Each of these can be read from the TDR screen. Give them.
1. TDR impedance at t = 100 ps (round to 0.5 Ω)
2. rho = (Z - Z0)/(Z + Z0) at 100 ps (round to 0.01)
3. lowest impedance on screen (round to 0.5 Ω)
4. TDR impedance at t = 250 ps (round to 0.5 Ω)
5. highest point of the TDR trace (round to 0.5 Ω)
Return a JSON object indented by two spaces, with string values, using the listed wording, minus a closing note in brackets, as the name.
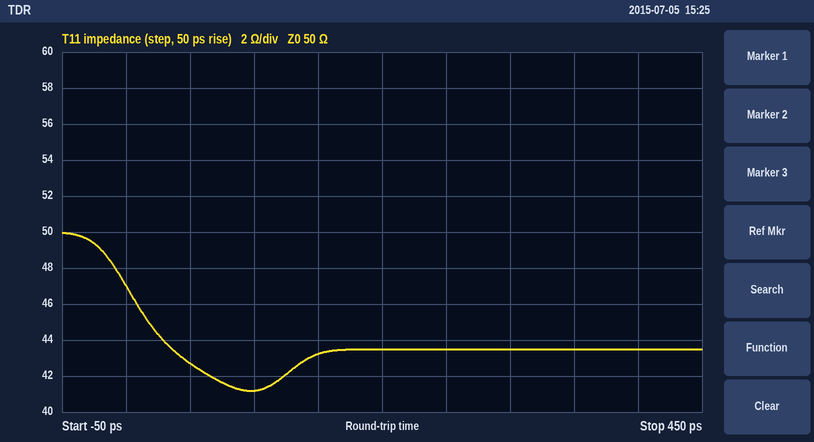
{
  "TDR impedance at t = 100 ps": "41.0 Ω",
  "rho = (Z - Z0)/(Z + Z0) at 100 ps": "-0.10",
  "lowest impedance on screen": "41.0 Ω",
  "TDR impedance at t = 250 ps": "43.5 Ω",
  "highest point of the TDR trace": "50.0 Ω"
}
